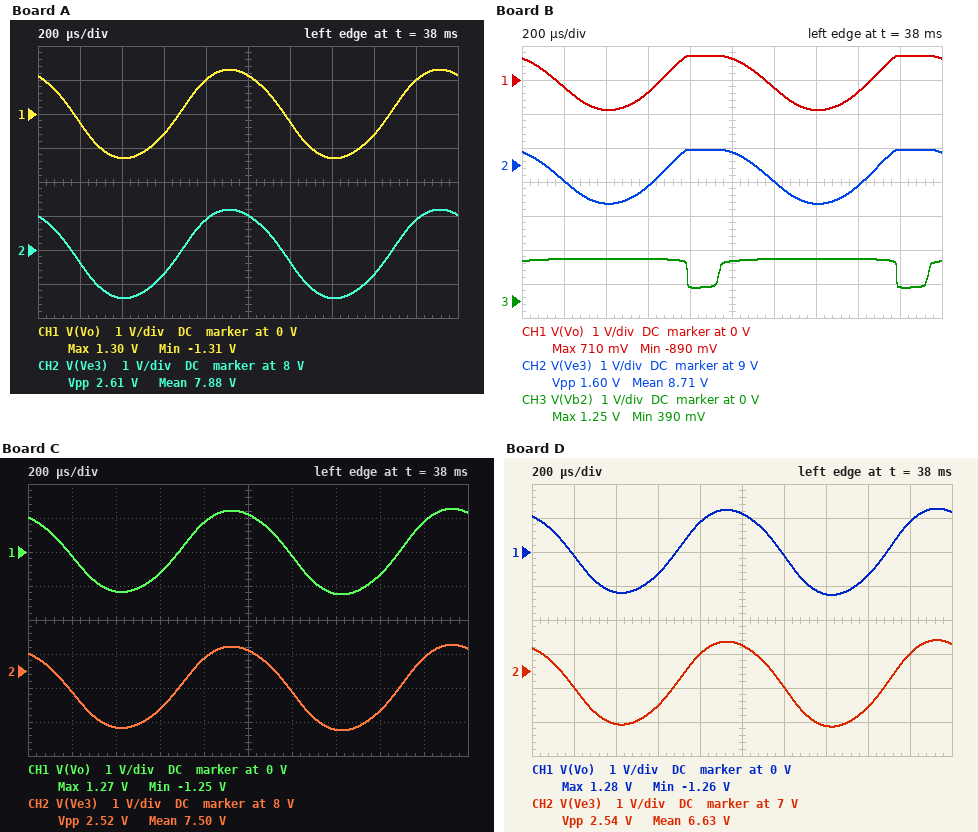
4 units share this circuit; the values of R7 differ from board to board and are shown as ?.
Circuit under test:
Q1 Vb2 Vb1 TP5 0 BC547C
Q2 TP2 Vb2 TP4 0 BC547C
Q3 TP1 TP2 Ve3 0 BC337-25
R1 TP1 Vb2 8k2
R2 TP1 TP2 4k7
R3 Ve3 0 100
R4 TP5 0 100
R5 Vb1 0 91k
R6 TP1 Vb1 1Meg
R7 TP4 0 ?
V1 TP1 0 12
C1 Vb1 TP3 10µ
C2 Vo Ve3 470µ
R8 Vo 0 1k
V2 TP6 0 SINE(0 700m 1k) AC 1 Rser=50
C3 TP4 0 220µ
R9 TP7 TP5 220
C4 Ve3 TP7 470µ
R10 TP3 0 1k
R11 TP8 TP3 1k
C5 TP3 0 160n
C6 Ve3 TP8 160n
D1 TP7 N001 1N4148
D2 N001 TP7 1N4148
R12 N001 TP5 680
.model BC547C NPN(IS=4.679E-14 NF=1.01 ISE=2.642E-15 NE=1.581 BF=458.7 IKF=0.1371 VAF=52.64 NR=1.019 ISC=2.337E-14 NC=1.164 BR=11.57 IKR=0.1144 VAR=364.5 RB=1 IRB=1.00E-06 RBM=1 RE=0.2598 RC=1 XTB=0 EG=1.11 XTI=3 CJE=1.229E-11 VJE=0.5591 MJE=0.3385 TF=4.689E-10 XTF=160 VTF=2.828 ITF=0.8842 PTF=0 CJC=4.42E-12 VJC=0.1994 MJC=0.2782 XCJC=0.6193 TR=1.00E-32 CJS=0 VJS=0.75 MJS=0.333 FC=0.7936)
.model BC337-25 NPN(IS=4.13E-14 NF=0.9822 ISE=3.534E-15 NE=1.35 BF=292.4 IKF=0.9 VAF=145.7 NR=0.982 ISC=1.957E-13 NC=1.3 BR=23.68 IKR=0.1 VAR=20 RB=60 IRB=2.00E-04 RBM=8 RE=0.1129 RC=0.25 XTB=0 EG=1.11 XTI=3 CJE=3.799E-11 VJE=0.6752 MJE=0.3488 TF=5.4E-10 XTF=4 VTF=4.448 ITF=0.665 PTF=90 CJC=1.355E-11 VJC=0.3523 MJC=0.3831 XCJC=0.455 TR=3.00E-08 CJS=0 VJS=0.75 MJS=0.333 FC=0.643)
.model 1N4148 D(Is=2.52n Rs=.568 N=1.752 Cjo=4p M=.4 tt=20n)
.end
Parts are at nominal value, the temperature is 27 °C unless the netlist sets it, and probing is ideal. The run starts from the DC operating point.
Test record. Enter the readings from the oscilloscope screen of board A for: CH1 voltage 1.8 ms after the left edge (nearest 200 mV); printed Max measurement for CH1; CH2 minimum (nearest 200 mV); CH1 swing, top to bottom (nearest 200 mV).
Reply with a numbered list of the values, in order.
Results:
1. 1.0 V
2. 1.30 V
3. 6.6 V
4. 2.6 V
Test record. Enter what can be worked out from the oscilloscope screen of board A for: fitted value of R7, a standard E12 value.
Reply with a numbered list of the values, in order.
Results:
1. 1.5 kΩ
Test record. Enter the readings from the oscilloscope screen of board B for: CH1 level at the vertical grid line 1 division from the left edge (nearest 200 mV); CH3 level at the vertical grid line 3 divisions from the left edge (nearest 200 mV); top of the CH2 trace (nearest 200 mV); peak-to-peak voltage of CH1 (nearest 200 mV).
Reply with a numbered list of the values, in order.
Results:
1. -200 mV
2. 1.2 V
3. 9.4 V
4. 1.6 V
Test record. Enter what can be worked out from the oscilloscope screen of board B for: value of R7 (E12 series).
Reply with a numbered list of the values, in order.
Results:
1. 3.3 kΩ
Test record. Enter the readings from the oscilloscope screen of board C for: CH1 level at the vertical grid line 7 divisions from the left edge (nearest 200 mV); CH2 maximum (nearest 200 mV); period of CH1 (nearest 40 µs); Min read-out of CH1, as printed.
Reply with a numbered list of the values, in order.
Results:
1. -1.2 V
2. 8.8 V
3. 1.00 ms
4. -1.25 V
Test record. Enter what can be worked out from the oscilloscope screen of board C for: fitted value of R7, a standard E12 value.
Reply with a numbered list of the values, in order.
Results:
1. 1.2 kΩ
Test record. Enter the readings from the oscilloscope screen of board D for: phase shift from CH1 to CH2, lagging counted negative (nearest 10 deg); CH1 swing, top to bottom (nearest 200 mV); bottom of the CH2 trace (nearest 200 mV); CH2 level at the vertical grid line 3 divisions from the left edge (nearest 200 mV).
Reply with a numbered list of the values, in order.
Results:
1. 0 deg
2. 2.6 V
3. 5.4 V
4. 6.0 V
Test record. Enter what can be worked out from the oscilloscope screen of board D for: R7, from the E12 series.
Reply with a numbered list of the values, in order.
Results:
1. 820 Ω
